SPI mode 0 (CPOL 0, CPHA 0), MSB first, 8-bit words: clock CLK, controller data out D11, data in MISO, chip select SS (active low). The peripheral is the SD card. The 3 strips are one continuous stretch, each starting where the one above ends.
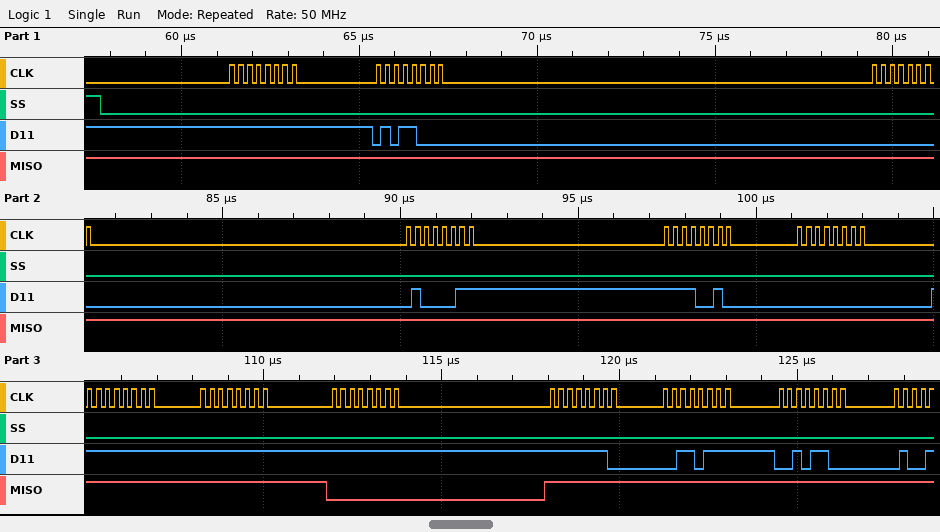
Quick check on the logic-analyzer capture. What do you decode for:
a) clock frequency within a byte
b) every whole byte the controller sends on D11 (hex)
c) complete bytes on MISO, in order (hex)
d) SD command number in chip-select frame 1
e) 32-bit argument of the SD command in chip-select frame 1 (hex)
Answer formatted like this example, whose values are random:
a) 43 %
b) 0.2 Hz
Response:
a) 4 MHz
b) FF 58 00 43 F2 00 FF FF FF FE 37 2C
c) FF FF FF FF FF FF FF FF 00 FF FF FF
d) CMD24
e) 0x0043F200
